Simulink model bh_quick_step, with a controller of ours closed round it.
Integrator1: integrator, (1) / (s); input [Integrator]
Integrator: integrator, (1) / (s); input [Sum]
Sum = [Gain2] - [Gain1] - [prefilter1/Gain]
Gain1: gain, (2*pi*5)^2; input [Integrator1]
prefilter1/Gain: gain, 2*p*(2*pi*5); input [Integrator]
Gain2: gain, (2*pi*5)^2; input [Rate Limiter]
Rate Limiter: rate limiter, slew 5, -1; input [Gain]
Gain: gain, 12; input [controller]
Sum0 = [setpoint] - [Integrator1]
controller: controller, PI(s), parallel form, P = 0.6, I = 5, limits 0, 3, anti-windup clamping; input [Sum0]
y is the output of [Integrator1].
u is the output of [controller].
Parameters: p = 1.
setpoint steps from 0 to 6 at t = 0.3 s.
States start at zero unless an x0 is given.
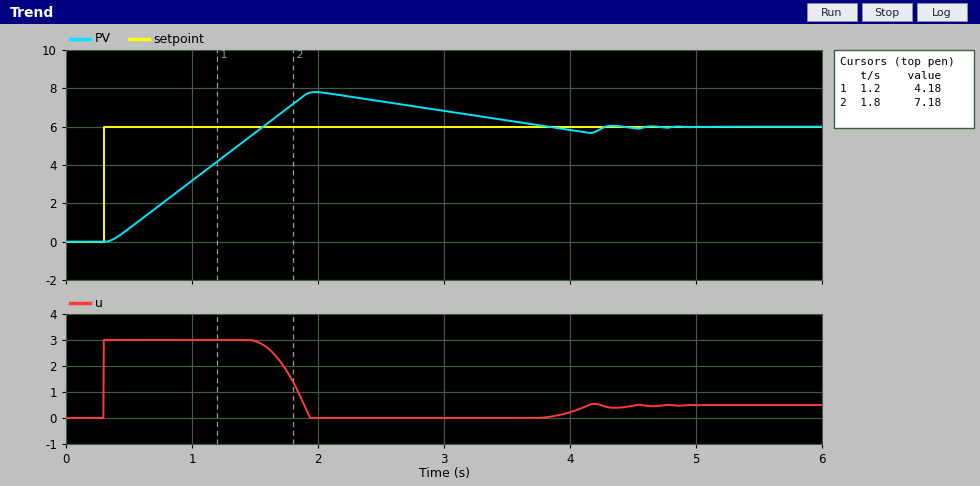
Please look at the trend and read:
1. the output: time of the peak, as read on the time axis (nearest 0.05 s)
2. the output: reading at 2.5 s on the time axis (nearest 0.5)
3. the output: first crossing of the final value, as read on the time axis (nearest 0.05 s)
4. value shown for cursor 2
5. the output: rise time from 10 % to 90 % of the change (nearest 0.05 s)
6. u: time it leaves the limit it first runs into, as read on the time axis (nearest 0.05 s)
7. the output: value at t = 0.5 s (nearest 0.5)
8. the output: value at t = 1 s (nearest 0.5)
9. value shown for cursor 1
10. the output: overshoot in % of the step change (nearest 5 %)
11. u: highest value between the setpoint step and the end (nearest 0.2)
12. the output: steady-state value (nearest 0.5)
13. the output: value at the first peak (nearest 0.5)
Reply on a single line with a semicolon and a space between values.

2.00 s; 7.5; 1.55 s; 7.18; 0.95 s; 1.50 s; 0.5; 3.0; 4.18; 30 %; 3.0; 6.0; 8.0
